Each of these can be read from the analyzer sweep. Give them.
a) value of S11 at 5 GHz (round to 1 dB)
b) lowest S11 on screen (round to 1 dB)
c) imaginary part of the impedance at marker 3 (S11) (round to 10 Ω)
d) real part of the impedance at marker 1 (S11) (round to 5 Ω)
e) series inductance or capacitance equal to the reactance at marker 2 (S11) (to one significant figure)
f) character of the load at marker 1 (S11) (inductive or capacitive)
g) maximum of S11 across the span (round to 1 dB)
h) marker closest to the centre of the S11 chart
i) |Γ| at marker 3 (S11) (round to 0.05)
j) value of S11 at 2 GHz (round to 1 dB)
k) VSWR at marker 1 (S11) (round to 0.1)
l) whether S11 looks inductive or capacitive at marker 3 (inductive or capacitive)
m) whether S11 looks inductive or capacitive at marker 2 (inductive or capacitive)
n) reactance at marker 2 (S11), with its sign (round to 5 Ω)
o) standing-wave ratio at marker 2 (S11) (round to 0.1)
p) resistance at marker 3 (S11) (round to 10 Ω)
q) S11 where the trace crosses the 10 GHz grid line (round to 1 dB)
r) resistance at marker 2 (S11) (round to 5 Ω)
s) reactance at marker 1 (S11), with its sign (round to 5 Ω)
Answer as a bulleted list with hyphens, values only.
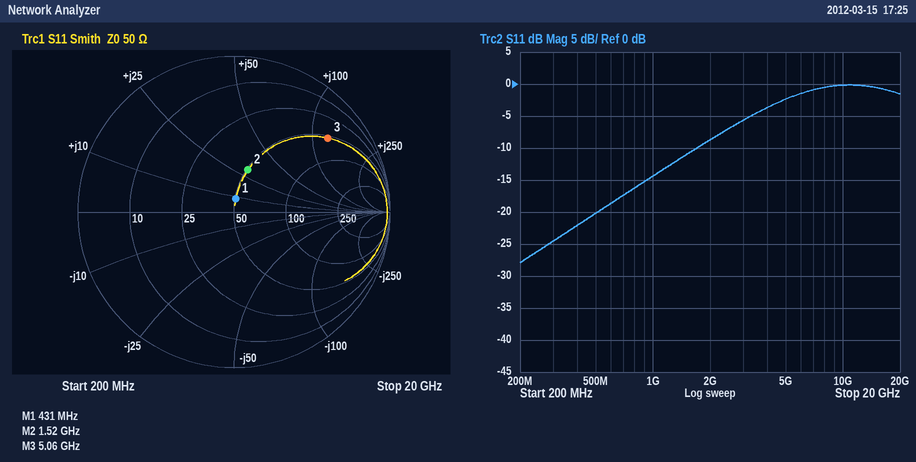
- -2 dB
- -28 dB
- +120 Ω
- 50 Ω
- 3 nH
- inductive
- 0 dB
- marker 1
- 0.75
- -9 dB
- 1.2
- inductive
- inductive
- +30 Ω
- 1.8
- 50 Ω
- 0 dB
- 50 Ω
- +10 Ω
